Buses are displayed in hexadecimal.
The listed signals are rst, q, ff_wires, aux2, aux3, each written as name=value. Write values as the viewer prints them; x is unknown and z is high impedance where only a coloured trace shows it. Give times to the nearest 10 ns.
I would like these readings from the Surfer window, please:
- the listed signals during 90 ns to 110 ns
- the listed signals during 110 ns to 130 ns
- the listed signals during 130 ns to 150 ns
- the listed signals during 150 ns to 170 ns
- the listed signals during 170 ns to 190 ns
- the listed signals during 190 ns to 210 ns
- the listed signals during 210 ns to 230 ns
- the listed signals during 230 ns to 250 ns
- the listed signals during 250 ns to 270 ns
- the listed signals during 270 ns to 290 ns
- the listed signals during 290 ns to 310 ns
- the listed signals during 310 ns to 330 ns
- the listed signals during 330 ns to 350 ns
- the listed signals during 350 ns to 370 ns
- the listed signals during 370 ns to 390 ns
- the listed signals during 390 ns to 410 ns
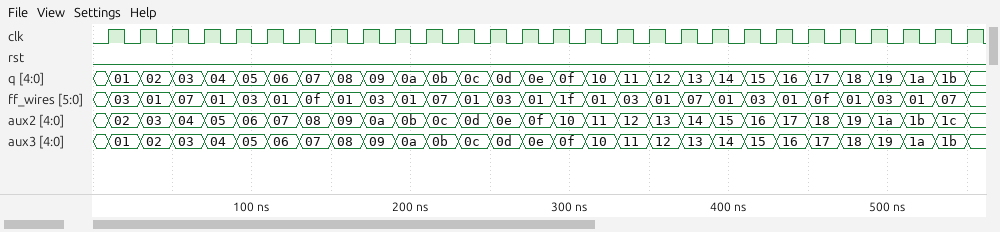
rst=0, q=05, ff_wires=03, aux2=06, aux3=05
rst=0, q=06, ff_wires=01, aux2=07, aux3=06
rst=0, q=07, ff_wires=0f, aux2=08, aux3=07
rst=0, q=08, ff_wires=01, aux2=09, aux3=08
rst=0, q=09, ff_wires=03, aux2=0a, aux3=09
rst=0, q=0a, ff_wires=01, aux2=0b, aux3=0a
rst=0, q=0b, ff_wires=07, aux2=0c, aux3=0b
rst=0, q=0c, ff_wires=01, aux2=0d, aux3=0c
rst=0, q=0d, ff_wires=03, aux2=0e, aux3=0d
rst=0, q=0e, ff_wires=01, aux2=0f, aux3=0e
rst=0, q=0f, ff_wires=1f, aux2=10, aux3=0f
rst=0, q=10, ff_wires=01, aux2=11, aux3=10
rst=0, q=11, ff_wires=03, aux2=12, aux3=11
rst=0, q=12, ff_wires=01, aux2=13, aux3=12
rst=0, q=13, ff_wires=07, aux2=14, aux3=13
rst=0, q=14, ff_wires=01, aux2=15, aux3=14
